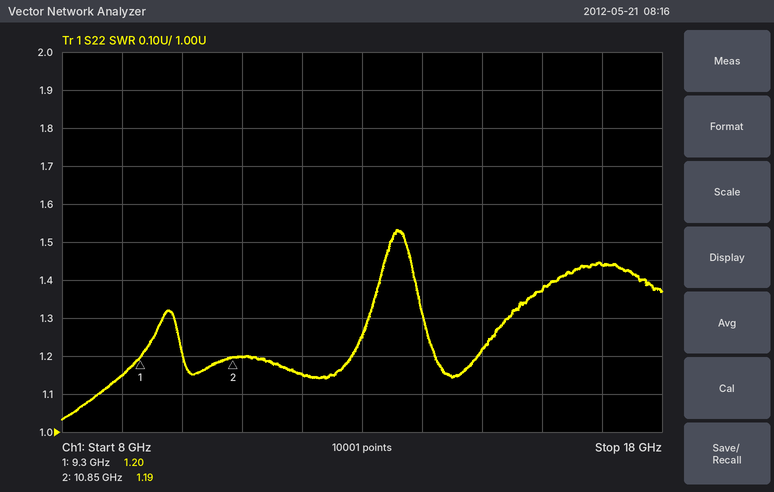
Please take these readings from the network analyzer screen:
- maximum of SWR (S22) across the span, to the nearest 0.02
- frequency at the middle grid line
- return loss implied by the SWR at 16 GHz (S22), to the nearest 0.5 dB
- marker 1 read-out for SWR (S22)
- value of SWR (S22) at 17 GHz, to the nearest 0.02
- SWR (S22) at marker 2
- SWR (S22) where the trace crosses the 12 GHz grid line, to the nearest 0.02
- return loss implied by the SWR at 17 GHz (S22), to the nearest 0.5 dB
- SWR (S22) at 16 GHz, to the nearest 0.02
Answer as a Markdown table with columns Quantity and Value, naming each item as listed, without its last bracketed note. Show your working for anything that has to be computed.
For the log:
| Quantity | Value |
|---|---|
| maximum of SWR (S22) across the span, to the nearest 0.02 | 1.54 |
| frequency at the middle grid line | 13 GHz |
| return loss implied by the SWR at 16 GHz (S22), to the nearest 0.5 dB | −20 log10((1.38 − 1)/(1.38 + 1)) ≈ 15.9 dB, so 16.0 dB to the nearest 0.5 dB |
| marker 1 read-out for SWR | 1.20 |
| value of SWR (S22) at 17 GHz, to the nearest 0.02 | 1.44 |
| SWR (S22) at marker 2 | 1.19 |
| SWR (S22) where the trace crosses the 12 GHz grid line, to the nearest 0.02 | 1.16 |
| return loss implied by the SWR at 17 GHz (S22), to the nearest 0.5 dB | −20 log10((1.44 − 1)/(1.44 + 1)) ≈ 14.9 dB, so 15.0 dB to the nearest 0.5 dB |
| SWR (S22) at 16 GHz, to the nearest 0.02 | 1.38 |
